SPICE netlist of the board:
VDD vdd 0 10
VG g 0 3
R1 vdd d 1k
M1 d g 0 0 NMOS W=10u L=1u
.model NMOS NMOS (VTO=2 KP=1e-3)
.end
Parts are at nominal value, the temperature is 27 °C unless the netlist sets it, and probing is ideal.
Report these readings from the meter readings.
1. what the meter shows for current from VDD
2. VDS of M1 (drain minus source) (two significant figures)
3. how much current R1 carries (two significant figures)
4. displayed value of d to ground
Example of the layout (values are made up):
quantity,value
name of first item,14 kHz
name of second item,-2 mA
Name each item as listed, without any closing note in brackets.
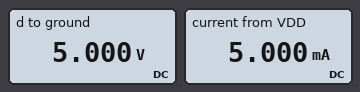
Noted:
quantity,value
what the meter shows for current from VDD,5.000 mA
VDS of M1 (drain minus source),5.0 V
how much current R1 carries,5.0 mA
displayed value of d to ground,5.000 V
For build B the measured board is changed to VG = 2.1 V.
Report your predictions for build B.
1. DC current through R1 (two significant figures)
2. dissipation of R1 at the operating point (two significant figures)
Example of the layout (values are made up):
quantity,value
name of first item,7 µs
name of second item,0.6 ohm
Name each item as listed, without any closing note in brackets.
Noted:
quantity,value
DC current through R1,50 µA
dissipation of R1 at the operating point,2.5 µW
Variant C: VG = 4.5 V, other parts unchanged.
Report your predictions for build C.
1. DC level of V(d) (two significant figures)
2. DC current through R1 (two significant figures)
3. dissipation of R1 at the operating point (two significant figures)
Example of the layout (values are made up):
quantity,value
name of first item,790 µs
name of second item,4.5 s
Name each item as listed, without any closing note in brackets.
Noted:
quantity,value
DC level of V(d),420 mV
DC current through R1,9.6 mA
dissipation of R1 at the operating point,92 mW
